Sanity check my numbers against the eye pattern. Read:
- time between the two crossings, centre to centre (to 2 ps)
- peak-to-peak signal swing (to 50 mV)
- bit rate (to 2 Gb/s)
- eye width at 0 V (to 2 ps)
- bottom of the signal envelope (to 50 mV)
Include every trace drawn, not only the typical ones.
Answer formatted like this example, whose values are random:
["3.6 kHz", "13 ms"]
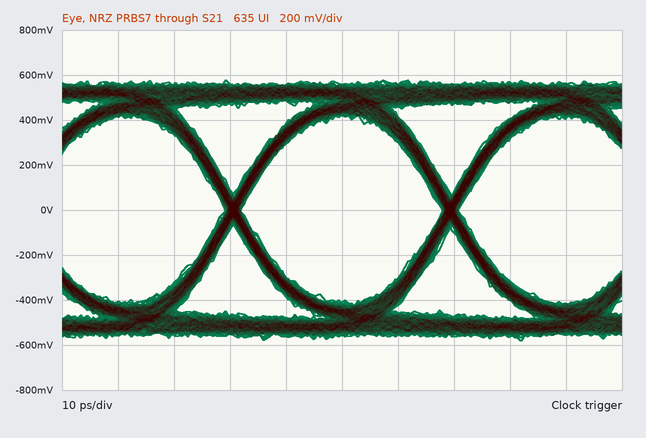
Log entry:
["38 ps", "1.15 V", "26 Gb/s", "36 ps", "-600 mV"]
